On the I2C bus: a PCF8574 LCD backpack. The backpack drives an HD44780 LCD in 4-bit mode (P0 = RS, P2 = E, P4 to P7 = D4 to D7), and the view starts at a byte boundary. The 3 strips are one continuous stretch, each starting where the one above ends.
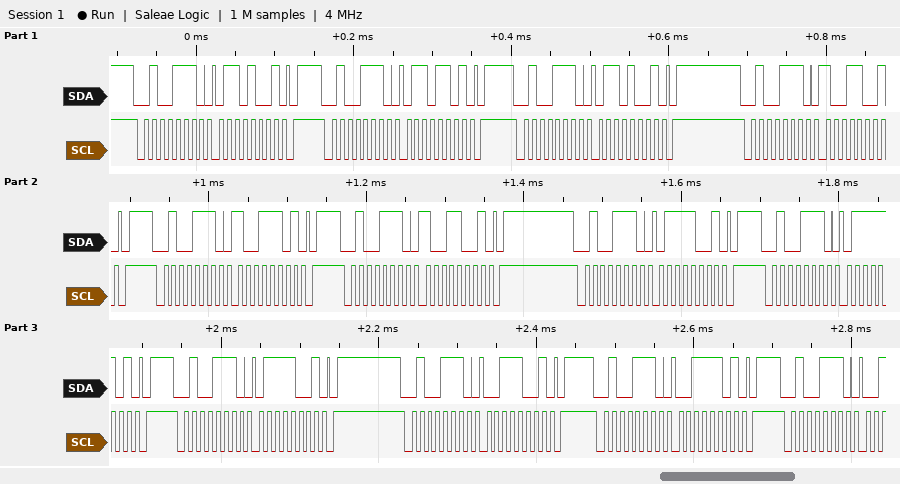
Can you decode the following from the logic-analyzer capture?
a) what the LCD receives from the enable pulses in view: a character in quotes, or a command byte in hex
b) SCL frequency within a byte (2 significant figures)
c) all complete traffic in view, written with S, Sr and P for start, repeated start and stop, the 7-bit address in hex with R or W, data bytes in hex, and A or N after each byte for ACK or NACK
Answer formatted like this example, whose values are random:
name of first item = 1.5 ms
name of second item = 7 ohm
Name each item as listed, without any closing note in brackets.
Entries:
what the LCD receives from the enable pulses in view: a character in quotes, or a command byte in hex = 'i'
SCL frequency within a byte = 100 kHz
all complete traffic in view, written with S, Sr and P for start, repeated start and stop, the 7-bit address in hex with R or W, data bytes in hex, and A or N after each byte for ACK or NACK = S 27W A 69 A P S 27W A 6D A P S 27W A 69 A P S 27W A 99 A P S 27W A 9D A P S 27W A 99 A P S 27W A 79 A P S 27W A 7D A P S 27W A 79 A P S 27W A 39 A P S 27W A 3D A P S 27W A
